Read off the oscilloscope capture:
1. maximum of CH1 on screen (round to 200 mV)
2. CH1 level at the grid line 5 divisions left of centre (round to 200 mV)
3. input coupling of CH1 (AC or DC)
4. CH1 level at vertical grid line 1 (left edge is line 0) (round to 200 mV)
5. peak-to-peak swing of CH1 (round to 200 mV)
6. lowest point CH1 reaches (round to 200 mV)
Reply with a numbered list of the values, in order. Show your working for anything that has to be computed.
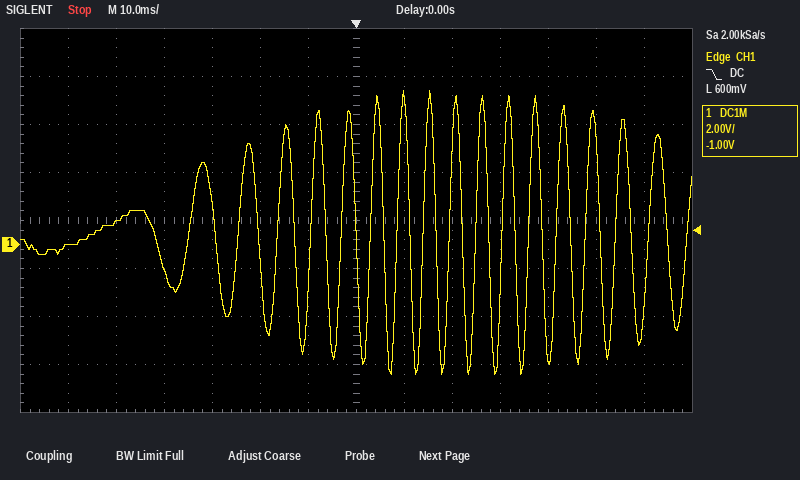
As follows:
1. 6.4 V
2. 1.0 V
3. DC
4. 0.0 V
5. 6.4 V − (-5.4 V) = 11.8 V
6. -5.4 V
